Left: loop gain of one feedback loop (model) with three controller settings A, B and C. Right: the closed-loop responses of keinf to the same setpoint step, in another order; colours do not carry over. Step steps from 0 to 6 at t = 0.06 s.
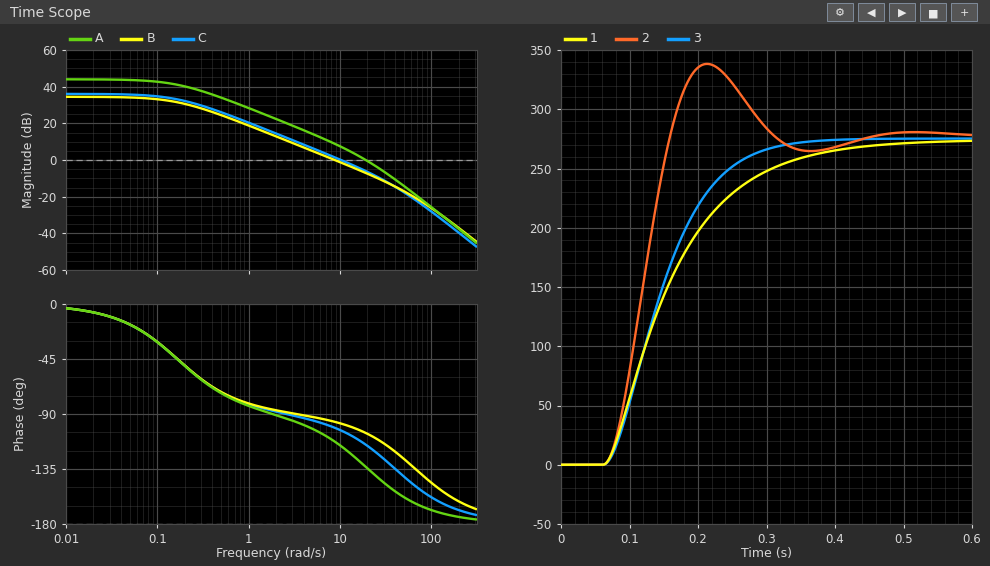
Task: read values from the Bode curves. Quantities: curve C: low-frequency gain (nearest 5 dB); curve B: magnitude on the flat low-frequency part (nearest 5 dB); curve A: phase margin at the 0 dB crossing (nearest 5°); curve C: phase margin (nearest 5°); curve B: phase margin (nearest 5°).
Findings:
35 dB
35 dB
45°
75°
85°
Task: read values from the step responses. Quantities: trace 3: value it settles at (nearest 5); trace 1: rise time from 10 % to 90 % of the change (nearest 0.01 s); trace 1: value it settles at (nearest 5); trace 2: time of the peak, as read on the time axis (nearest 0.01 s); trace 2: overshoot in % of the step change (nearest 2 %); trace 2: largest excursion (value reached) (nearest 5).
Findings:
275
0.21 s
275
0.21 s
22 %
340
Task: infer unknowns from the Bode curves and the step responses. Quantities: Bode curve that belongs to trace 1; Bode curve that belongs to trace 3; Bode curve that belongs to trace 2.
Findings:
B
C
A
